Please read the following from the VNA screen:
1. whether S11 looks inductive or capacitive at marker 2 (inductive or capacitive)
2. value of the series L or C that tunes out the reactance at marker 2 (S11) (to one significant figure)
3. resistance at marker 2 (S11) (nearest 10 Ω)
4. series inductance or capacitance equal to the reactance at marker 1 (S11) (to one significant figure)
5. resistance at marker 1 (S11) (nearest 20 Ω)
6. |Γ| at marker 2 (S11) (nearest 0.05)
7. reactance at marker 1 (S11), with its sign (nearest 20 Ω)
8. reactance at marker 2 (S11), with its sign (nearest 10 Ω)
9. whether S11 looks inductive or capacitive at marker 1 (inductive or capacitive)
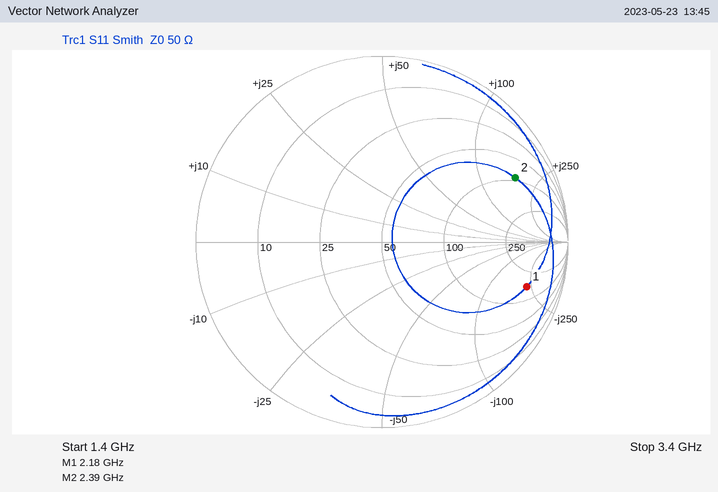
inductive
400 fF
90 Ω
300 fF
160 Ω
0.80
-220 Ω
+170 Ω
capacitive
